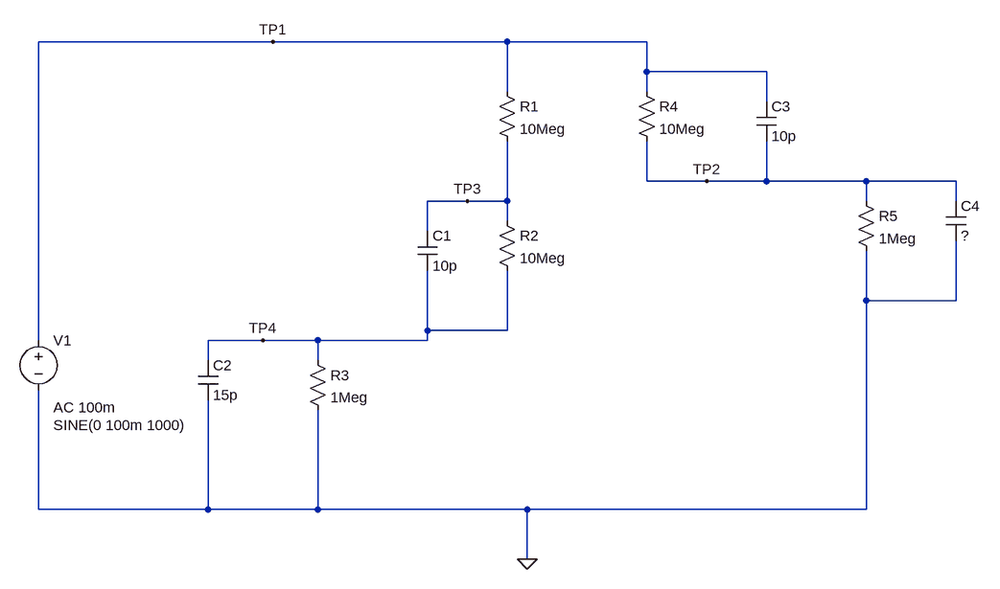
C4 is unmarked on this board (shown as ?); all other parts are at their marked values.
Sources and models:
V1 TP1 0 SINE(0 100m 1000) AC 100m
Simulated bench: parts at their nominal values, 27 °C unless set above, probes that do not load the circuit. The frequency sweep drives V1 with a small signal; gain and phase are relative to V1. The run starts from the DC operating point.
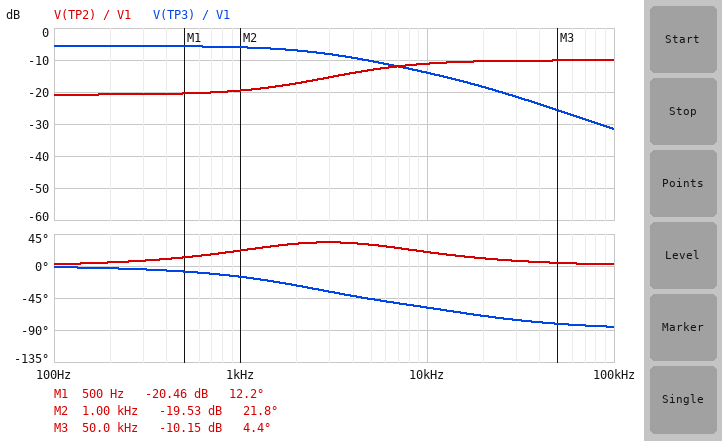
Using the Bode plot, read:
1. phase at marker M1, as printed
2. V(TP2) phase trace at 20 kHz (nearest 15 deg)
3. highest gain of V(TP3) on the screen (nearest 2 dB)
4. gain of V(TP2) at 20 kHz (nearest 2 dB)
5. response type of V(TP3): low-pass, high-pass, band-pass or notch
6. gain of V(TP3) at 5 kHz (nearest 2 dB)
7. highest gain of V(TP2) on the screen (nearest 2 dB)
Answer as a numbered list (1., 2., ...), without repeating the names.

1. 12.2 deg
2. 15 deg
3. -6 dB
4. -10 dB
5. low-pass
6. -10 dB
7. -10 dB
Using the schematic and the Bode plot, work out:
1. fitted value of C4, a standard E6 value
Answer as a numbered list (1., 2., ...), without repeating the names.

1. 22 pF
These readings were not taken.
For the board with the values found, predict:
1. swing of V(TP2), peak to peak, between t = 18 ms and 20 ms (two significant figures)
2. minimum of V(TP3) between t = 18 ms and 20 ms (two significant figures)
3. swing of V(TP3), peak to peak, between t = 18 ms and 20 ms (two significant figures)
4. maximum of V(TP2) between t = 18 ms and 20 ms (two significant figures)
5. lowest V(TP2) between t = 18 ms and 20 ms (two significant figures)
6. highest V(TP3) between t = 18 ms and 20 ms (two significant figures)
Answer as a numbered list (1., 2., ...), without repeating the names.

1. 21 mV
2. -50 mV
3. 100 mV
4. 11 mV
5. -11 mV
6. 50 mV
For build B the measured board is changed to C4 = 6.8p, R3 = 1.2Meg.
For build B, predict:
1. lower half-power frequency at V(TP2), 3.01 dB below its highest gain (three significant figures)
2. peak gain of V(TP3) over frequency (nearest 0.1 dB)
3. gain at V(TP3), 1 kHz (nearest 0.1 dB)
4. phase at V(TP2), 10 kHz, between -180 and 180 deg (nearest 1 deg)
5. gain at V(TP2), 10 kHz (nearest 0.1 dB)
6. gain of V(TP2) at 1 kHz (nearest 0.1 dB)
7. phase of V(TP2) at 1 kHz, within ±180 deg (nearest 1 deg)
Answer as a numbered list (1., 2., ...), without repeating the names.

1. 10.2 kHz
2. -5.5 dB
3. -5.9 dB
4. 37 deg
5. -7.6 dB
6. -19.4 dB
7. 27 deg
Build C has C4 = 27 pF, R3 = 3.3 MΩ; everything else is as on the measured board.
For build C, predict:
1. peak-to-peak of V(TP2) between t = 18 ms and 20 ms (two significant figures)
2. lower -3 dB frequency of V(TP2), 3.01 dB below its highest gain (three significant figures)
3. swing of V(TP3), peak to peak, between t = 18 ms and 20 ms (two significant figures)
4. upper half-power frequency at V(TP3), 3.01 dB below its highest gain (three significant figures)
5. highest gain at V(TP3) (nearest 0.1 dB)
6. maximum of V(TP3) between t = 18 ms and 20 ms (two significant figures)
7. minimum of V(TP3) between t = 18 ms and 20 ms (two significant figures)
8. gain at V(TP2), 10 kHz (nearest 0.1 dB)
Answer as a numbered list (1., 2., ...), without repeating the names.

1. 21 mV
2. 4.16 kHz
3. 110 mV
4. 4.35 kHz
5. -4.9 dB
6. 55 mV
7. -55 mV
8. -12.1 dB
